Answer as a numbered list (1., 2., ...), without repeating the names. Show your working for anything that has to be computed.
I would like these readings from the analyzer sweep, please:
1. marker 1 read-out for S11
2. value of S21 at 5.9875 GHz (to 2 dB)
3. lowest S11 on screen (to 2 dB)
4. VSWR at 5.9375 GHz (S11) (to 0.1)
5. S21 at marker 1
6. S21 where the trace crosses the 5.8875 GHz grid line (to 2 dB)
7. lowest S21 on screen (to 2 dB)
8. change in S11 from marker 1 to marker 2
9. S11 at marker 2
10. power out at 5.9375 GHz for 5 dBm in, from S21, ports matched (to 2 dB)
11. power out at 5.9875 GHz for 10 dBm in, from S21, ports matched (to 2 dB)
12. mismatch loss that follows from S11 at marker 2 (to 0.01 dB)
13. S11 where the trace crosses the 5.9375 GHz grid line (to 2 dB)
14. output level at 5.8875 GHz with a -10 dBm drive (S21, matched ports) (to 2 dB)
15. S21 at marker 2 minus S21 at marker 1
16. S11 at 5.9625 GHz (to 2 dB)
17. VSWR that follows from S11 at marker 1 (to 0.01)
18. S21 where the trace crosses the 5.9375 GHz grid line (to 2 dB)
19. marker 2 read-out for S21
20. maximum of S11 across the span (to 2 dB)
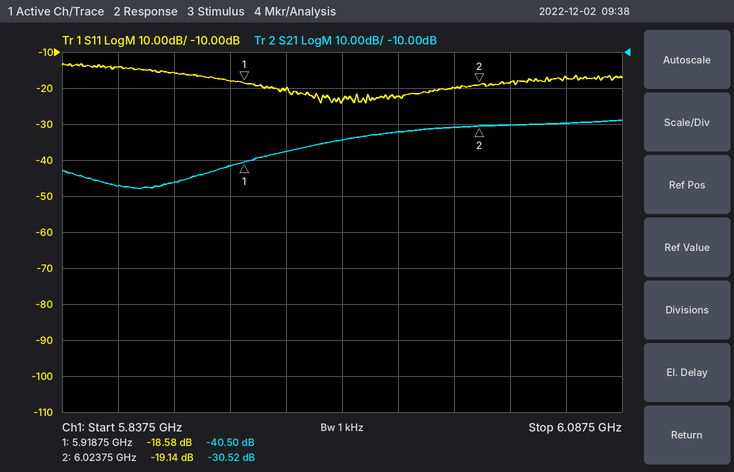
1. -18.58 dB
2. -32 dB
3. -24 dB
4. |Γ| = 10^(-20/20) = 0.1000; VSWR = (1 + 0.1000)/(1 − 0.1000) ≈ 1.2
5. -40.50 dB
6. -46 dB
7. -48 dB
8. -19.14 − (-18.58) = -0.56 dB
9. -19.14 dB
10. 5 dBm + (-38 dB) = -32 dBm
11. 10 dBm + (-32 dB) = -22 dBm
12. −10 log10(1 − 10^(-19.14/10)) ≈ 0.05 dB
13. -20 dB
14. -10 dBm + (-46 dB) = -56 dBm
15. -30.52 − (-40.5) = 9.98 dB
16. -24 dB
17. (1 + 0.1178)/(1 − 0.1178) ≈ 1.27
18. -38 dB
19. -30.52 dB
20. -14 dB
